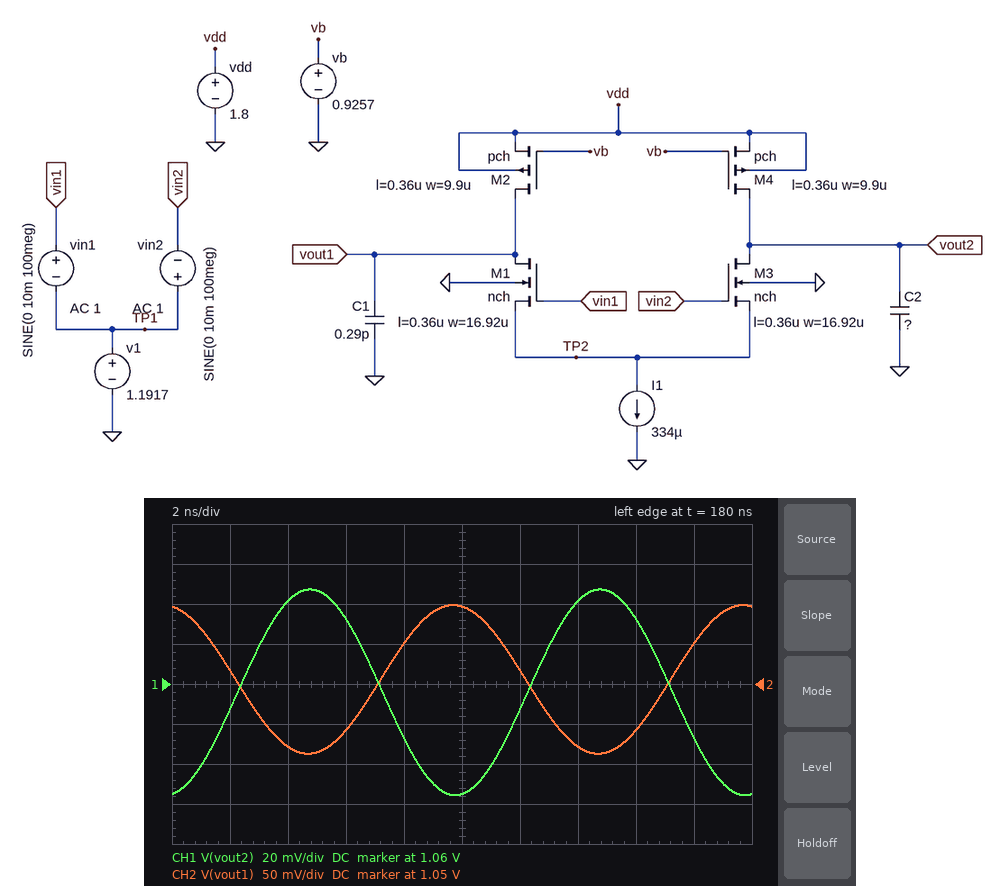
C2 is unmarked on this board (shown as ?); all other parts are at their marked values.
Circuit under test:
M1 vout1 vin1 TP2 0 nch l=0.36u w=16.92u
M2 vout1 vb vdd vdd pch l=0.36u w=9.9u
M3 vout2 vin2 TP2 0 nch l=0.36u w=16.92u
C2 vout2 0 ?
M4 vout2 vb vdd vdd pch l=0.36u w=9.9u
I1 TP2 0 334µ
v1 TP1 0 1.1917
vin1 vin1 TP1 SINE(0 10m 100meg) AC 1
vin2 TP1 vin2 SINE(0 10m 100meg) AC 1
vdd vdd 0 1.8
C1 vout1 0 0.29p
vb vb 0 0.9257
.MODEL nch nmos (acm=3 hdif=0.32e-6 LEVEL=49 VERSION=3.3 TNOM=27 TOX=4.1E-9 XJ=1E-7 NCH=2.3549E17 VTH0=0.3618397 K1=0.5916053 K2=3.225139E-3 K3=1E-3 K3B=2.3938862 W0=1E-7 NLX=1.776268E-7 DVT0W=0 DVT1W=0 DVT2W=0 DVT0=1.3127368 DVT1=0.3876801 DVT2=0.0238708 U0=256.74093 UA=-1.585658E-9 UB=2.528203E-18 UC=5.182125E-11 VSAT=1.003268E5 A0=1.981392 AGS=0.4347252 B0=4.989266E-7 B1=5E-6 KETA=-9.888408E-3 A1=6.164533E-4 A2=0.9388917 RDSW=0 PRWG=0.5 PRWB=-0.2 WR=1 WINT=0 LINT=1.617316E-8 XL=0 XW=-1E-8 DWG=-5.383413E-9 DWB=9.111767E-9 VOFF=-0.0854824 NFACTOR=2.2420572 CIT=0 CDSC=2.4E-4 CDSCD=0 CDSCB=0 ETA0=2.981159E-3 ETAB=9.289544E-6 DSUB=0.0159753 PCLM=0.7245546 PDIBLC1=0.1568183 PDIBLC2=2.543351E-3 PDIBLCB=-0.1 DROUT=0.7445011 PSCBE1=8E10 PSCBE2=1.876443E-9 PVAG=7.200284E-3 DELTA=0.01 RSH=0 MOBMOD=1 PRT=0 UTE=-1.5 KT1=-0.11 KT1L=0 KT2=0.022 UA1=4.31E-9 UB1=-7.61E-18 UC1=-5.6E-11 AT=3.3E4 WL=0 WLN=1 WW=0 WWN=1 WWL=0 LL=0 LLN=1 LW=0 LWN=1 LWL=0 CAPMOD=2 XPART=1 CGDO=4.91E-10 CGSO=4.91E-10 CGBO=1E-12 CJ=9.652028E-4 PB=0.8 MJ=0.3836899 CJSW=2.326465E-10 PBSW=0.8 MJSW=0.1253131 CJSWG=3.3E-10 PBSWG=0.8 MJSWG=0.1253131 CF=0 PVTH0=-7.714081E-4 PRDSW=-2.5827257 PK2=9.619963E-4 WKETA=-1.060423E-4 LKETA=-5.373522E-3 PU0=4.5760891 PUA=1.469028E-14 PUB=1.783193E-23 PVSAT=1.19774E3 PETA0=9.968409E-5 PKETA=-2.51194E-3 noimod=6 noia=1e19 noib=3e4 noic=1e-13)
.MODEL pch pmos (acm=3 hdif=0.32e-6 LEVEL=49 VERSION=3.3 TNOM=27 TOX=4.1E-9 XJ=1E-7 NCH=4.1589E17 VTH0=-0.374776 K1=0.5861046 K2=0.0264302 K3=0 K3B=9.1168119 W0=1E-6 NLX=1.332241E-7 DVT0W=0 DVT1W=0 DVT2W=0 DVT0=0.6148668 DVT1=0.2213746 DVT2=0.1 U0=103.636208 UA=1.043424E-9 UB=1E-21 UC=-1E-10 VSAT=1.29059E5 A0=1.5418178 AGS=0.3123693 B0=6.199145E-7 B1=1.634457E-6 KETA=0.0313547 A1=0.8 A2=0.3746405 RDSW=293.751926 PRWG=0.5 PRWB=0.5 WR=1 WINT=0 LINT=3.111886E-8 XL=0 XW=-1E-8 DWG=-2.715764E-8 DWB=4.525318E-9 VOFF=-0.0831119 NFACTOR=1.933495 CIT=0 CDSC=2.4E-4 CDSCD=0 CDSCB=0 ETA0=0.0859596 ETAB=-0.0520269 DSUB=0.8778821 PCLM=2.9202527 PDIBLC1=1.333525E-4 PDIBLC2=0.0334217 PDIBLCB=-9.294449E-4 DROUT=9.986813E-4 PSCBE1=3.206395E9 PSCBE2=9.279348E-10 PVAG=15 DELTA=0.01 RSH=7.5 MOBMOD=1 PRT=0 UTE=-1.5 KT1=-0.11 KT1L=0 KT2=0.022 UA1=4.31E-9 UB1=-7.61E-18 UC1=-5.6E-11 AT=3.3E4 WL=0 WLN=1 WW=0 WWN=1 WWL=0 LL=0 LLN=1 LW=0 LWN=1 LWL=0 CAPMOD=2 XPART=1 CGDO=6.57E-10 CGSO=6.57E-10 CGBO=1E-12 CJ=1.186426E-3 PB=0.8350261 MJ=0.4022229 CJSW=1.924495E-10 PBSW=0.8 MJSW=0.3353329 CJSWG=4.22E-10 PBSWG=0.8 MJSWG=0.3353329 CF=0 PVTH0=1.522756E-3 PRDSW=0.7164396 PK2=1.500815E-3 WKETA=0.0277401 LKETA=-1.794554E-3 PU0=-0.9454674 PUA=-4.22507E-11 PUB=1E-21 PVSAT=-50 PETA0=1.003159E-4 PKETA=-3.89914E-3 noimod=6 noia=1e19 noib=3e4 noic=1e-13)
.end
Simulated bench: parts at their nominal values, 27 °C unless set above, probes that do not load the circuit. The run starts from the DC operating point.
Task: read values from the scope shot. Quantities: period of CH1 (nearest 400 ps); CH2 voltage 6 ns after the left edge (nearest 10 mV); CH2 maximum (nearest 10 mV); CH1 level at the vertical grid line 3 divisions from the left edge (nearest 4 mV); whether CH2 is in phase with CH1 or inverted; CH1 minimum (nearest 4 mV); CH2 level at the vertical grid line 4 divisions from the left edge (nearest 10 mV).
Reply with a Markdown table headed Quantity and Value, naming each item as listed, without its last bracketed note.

| Quantity | Value |
|---|---|
| period of CH1 | 10.0 ns |
| CH2 voltage 6 ns after the left edge | 990 mV |
| CH2 maximum | 1.15 V |
| CH1 level at the vertical grid line 3 divisions from the left edge | 1.092 V |
| whether CH2 is in phase with CH1 or inverted | inverted |
| CH1 minimum | 1.004 V |
| CH2 level at the vertical grid line 4 divisions from the left edge | 1.10 V |
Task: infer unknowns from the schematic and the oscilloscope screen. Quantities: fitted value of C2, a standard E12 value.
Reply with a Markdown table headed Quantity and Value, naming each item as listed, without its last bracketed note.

| Quantity | Value |
|---|---|
| fitted value of C2, a standard E12 value | 560 fF |
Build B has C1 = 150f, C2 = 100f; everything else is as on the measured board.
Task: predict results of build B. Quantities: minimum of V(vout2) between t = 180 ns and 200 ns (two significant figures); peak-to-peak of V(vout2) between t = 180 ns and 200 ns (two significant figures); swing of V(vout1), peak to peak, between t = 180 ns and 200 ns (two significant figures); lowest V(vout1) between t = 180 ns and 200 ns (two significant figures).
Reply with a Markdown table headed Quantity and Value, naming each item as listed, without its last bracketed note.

| Quantity | Value |
|---|---|
| minimum of V(vout2) between t = 180 ns and 200 ns | 850 mV |
| peak-to-peak of V(vout2) between t = 180 ns and 200 ns | 400 mV |
| swing of V(vout1), peak to peak, between t = 180 ns and 200 ns | 300 mV |
| lowest V(vout1) between t = 180 ns and 200 ns | 900 mV |
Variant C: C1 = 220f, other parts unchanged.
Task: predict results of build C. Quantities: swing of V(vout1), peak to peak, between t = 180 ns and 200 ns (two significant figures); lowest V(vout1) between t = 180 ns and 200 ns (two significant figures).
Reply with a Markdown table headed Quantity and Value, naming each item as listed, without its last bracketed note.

| Quantity | Value |
|---|---|
| swing of V(vout1), peak to peak, between t = 180 ns and 200 ns | 230 mV |
| lowest V(vout1) between t = 180 ns and 200 ns | 940 mV |
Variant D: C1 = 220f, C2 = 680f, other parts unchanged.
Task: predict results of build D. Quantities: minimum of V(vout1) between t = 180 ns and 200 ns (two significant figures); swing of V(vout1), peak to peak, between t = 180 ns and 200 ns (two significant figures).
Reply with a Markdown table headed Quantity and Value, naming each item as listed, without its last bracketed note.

| Quantity | Value |
|---|---|
| minimum of V(vout1) between t = 180 ns and 200 ns | 940 mV |
| swing of V(vout1), peak to peak, between t = 180 ns and 200 ns | 230 mV |
